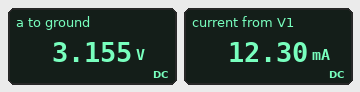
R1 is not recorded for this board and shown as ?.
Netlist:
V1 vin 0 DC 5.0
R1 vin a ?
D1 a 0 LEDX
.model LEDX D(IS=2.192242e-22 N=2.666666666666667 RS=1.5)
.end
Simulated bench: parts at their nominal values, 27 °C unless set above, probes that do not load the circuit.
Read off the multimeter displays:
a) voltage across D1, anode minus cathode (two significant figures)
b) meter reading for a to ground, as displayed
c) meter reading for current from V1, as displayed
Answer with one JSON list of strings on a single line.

["3.2 V", "3.155 V", "12.30 mA"]
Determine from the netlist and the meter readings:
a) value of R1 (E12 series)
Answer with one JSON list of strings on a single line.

["150 Ω"]
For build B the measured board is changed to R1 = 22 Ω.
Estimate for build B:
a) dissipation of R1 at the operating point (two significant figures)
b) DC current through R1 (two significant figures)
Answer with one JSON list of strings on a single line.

["120 mW", "74 mA"]
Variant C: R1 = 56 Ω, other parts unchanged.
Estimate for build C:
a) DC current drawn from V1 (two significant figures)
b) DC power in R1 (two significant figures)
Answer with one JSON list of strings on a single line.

["31 mA", "55 mW"]
